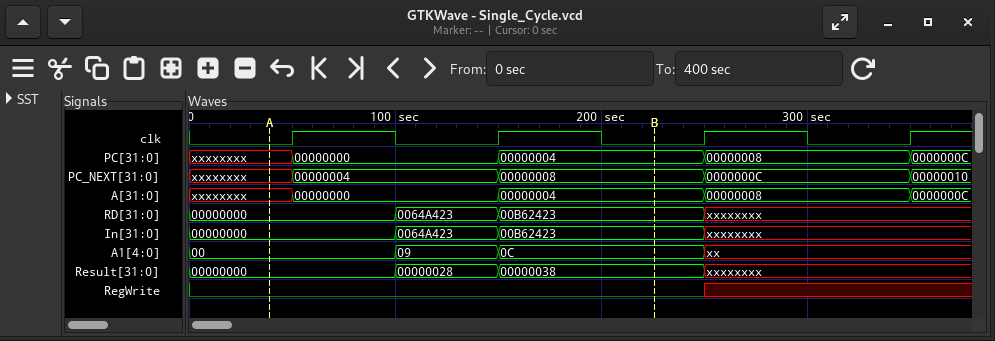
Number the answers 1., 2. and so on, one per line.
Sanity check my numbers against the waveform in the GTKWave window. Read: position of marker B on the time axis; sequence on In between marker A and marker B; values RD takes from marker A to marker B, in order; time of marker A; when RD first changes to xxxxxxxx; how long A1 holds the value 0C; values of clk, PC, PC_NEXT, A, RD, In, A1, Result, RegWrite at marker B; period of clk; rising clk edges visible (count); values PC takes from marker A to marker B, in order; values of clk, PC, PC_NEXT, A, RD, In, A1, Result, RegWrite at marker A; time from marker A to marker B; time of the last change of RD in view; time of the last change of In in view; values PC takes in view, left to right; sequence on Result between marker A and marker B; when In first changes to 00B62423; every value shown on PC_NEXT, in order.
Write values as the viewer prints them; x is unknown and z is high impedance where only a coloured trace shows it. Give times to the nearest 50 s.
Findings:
1. 250 s
2. 00000000, 0064A423, 00B62423
3. 00000000, 0064A423, 00B62423
4. 50 s
5. 250 s
6. 100 s
7. clk=0, PC=00000004, PC_NEXT=00000008, A=00000004, RD=00B62423, In=00B62423, A1=0C, Result=00000038, RegWrite=0
8. 100 s
9. 4
10. xxxxxxxx, 00000000, 00000004
11. clk=0, PC=xxxxxxxx, PC_NEXT=xxxxxxxx, A=xxxxxxxx, RD=00000000, In=00000000, A1=00, Result=00000000, RegWrite=0
12. 200 s
13. 250 s
14. 250 s
15. xxxxxxxx, 00000000, 00000004, 00000008, 0000000C
16. 00000000, 00000028, 00000038
17. 150 s
18. xxxxxxxx, 00000004, 00000008, 0000000C, 00000010
